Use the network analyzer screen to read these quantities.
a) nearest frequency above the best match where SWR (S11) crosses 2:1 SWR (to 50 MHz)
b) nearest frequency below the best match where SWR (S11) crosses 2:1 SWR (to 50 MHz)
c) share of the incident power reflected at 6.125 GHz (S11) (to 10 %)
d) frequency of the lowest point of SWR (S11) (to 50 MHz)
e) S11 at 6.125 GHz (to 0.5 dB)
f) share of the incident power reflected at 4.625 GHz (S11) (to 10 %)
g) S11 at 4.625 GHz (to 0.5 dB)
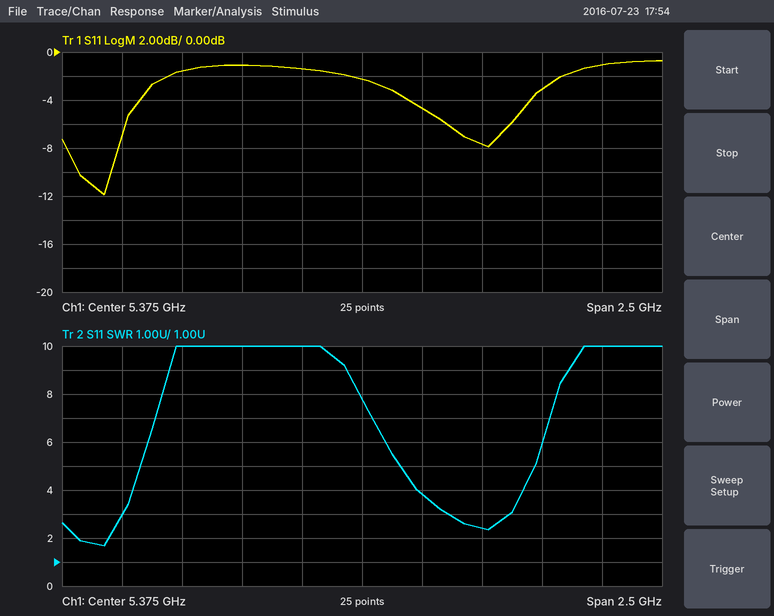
4.30 GHz
4.20 GHz
50 %
4.30 GHz
-3.0 dB
70 %
-1.5 dB
